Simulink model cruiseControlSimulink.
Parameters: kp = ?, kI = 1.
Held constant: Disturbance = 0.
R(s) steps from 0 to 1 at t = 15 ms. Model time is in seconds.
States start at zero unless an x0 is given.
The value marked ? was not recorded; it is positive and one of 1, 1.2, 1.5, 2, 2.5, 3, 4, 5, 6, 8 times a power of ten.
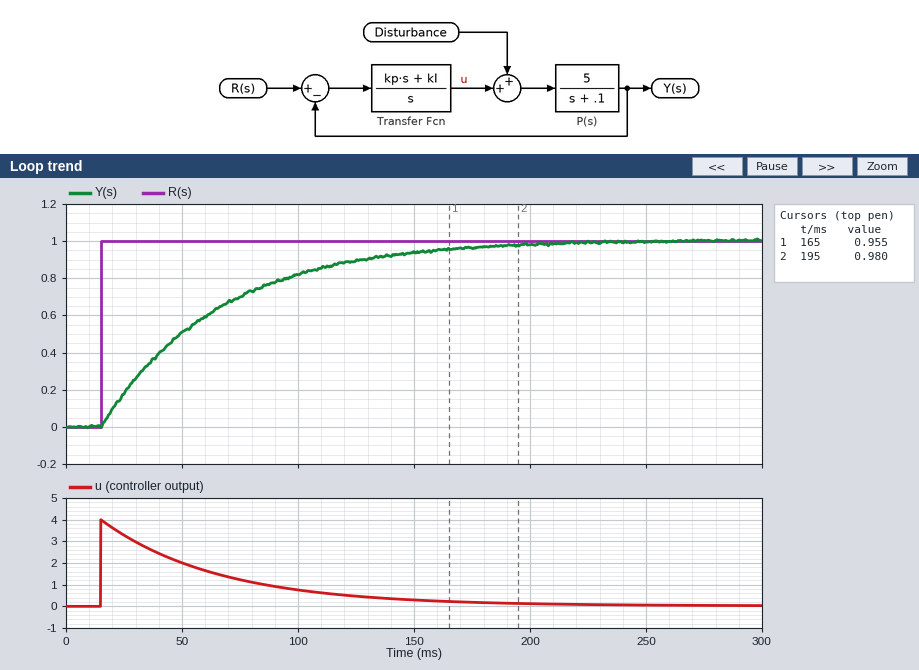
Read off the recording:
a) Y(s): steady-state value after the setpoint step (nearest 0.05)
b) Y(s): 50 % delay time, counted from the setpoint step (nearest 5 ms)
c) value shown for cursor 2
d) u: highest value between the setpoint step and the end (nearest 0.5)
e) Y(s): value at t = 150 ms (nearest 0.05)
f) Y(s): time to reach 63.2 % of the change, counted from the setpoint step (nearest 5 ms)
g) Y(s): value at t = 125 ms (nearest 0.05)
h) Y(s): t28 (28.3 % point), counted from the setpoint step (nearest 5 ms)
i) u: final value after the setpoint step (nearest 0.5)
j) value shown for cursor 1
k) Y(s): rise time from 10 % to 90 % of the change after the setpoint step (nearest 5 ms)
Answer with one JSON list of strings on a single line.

["1.00", "35 ms", "0.980", "4.0", "0.95", "50 ms", "0.90", "15 ms", "0.0", "0.955", "110 ms"]
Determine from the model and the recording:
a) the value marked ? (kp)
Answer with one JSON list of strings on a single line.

["4"]
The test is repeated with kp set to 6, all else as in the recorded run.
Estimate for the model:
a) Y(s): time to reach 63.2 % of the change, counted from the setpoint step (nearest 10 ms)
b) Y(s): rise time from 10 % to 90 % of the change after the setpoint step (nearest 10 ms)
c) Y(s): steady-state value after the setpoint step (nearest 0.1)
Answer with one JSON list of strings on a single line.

["30 ms", "70 ms", "1.0"]
